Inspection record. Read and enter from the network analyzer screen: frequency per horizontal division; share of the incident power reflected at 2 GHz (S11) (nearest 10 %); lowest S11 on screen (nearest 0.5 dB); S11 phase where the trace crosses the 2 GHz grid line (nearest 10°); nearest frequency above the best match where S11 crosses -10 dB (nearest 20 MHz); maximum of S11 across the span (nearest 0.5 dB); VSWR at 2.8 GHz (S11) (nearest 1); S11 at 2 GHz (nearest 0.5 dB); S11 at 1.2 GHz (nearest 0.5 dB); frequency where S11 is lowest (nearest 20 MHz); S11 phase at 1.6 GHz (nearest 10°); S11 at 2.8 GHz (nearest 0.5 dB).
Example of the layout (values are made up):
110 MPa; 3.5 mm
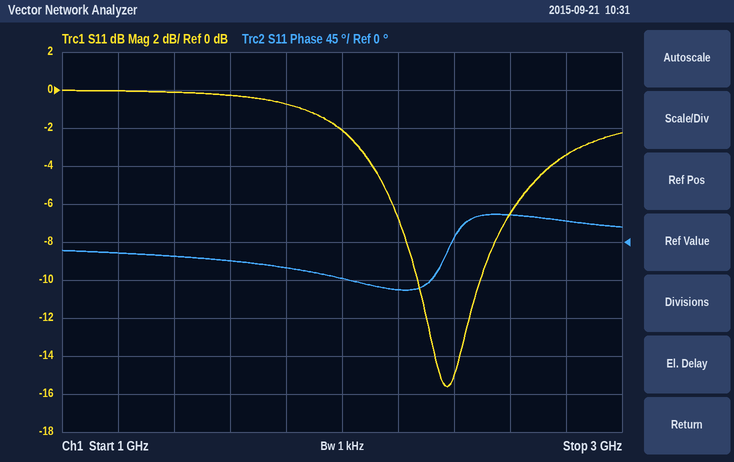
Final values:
200 MHz; 60 %; -15.5 dB; -40°; 2.50 GHz; 0.0 dB; 5; -2.0 dB; 0.0 dB; 2.38 GHz; -20°; -3.5 dB
